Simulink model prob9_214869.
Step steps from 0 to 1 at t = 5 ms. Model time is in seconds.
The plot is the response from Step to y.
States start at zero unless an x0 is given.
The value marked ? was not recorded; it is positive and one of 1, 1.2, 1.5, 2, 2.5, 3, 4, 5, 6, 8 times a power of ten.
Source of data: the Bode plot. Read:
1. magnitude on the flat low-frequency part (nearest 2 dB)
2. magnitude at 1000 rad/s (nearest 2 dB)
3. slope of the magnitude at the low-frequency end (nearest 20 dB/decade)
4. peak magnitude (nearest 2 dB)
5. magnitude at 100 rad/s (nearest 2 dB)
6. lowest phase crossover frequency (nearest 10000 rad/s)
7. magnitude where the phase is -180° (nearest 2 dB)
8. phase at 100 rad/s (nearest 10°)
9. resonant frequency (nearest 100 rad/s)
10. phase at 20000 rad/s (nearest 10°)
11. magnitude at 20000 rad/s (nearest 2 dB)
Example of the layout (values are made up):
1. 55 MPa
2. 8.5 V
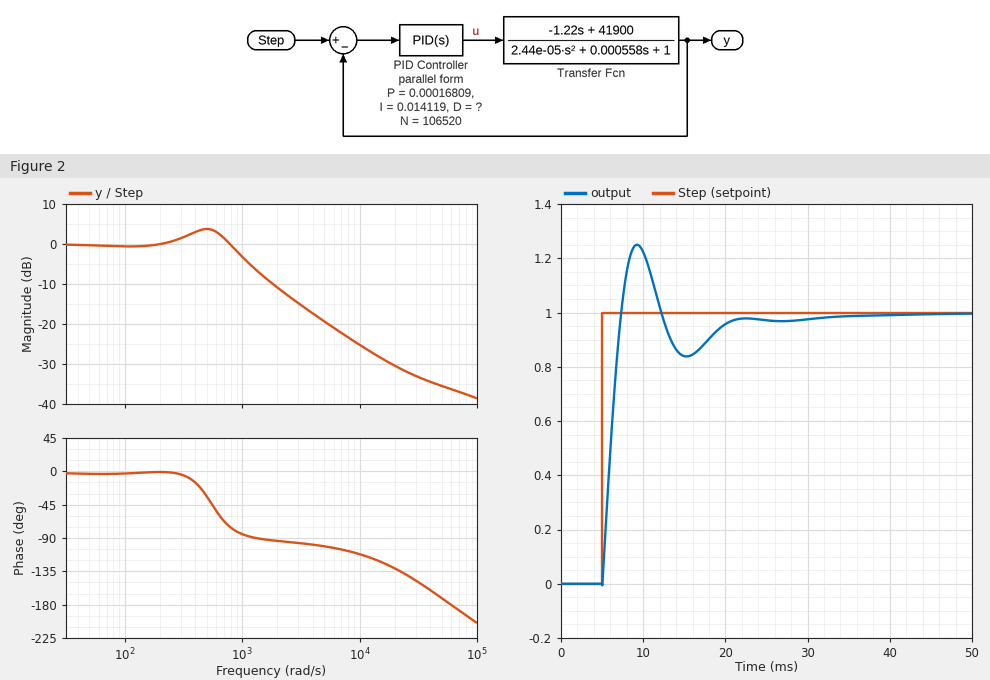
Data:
1. 0 dB
2. -4 dB
3. 0 dB/decade
4. 4 dB
5. 0 dB
6. 60000 rad/s
7. -36 dB
8. 0°
9. 500 rad/s
10. -130°
11. -30 dB
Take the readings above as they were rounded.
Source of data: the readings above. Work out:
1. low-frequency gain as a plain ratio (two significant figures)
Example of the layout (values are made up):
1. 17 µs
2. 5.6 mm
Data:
1. 1.0
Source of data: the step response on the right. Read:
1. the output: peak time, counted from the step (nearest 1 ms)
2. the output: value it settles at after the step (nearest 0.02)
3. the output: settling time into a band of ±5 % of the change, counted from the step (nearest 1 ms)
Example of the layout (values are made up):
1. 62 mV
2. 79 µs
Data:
1. 4 ms
2. 1.00
3. 15 ms
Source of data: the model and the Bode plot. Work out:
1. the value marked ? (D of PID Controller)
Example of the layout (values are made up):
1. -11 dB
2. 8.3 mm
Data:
1. 3e-07
